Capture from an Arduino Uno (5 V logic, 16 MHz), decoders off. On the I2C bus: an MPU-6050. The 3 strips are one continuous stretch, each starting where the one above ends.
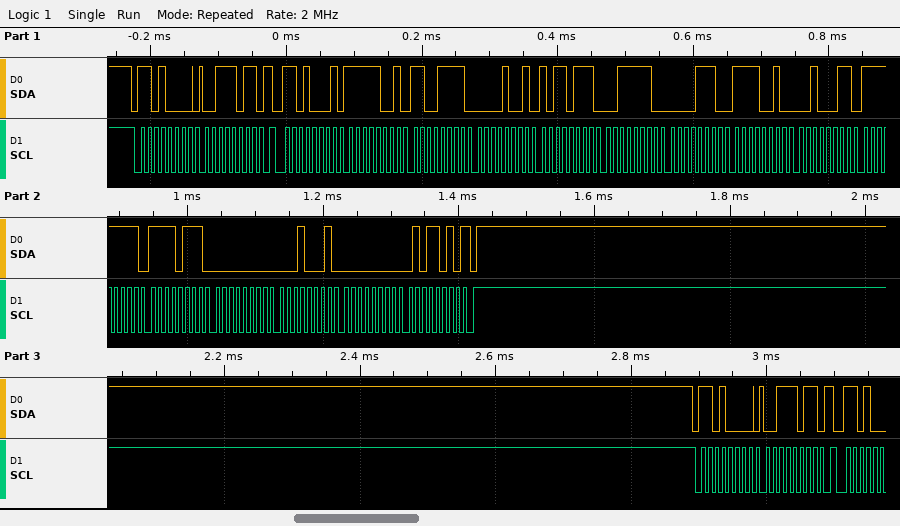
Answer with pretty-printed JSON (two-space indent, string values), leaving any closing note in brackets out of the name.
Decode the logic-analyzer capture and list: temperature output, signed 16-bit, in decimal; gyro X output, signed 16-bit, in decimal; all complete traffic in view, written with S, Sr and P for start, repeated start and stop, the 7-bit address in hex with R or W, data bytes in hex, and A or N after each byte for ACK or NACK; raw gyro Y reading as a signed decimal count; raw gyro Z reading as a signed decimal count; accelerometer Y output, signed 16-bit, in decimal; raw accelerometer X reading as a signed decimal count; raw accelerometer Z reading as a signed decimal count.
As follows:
{
  "temperature output, signed 16-bit, in decimal": "-3549",
  "gyro X output, signed 16-bit, in decimal": "-9",
  "all complete traffic in view, written with S, Sr and P for start, repeated start and stop, the 7-bit address in hex with R or W, data bytes in hex, and A or N after each byte for ACK or NACK": "S 68W A 3B A Sr 68R A F9 A CF A 09 A B7 A 3E A 0E A F2 A 23 A FF A F7 A 00 A 11 A 00 A 5A N P S 68W A 3B A",
  "raw gyro Y reading as a signed decimal count": "17",
  "raw gyro Z reading as a signed decimal count": "90",
  "accelerometer Y output, signed 16-bit, in decimal": "2487",
  "raw accelerometer X reading as a signed decimal count": "-1585",
  "raw accelerometer Z reading as a signed decimal count": "15886"
}
